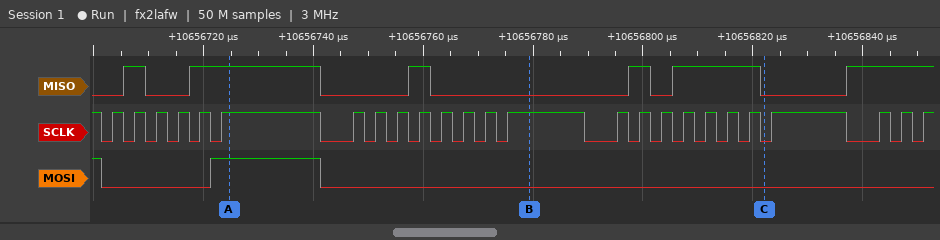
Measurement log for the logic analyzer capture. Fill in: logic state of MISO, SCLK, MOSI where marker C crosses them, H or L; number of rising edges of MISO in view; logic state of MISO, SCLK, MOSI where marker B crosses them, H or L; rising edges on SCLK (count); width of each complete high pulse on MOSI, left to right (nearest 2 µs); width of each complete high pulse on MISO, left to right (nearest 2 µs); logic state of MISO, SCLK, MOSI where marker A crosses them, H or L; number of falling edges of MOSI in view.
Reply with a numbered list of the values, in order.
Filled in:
1. MISO=L, SCLK=L, MOSI=L
2. 6
3. MISO=L, SCLK=H, MOSI=L
4. 25
5. 20 µs
6. 4 µs, 24 µs, 4 µs, 4 µs, 16 µs
7. MISO=H, SCLK=H, MOSI=H
8. 2
